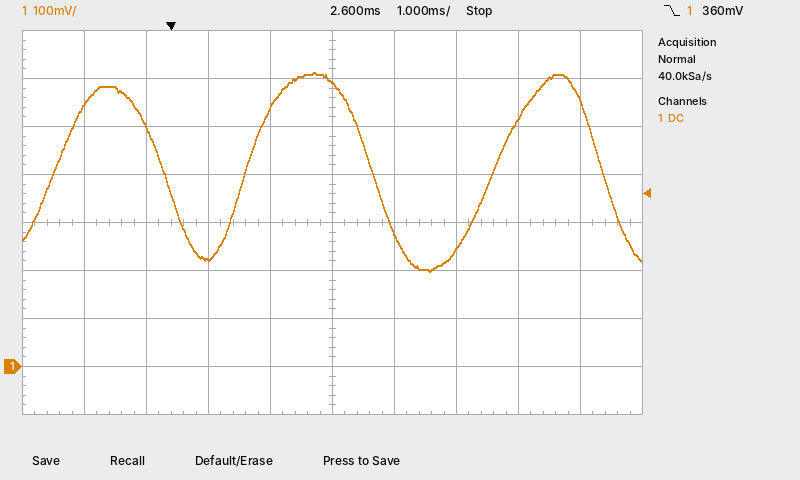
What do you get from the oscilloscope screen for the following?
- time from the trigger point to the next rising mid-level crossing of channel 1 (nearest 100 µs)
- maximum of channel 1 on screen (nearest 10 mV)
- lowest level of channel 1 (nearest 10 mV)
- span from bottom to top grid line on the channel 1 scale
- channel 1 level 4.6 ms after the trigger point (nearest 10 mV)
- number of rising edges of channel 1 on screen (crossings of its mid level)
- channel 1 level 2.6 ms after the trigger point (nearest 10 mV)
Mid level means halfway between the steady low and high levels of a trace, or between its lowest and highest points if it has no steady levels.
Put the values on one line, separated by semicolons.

1.2 ms; 610 mV; 200 mV; 800 mV; 240 mV; 3; 590 mV
